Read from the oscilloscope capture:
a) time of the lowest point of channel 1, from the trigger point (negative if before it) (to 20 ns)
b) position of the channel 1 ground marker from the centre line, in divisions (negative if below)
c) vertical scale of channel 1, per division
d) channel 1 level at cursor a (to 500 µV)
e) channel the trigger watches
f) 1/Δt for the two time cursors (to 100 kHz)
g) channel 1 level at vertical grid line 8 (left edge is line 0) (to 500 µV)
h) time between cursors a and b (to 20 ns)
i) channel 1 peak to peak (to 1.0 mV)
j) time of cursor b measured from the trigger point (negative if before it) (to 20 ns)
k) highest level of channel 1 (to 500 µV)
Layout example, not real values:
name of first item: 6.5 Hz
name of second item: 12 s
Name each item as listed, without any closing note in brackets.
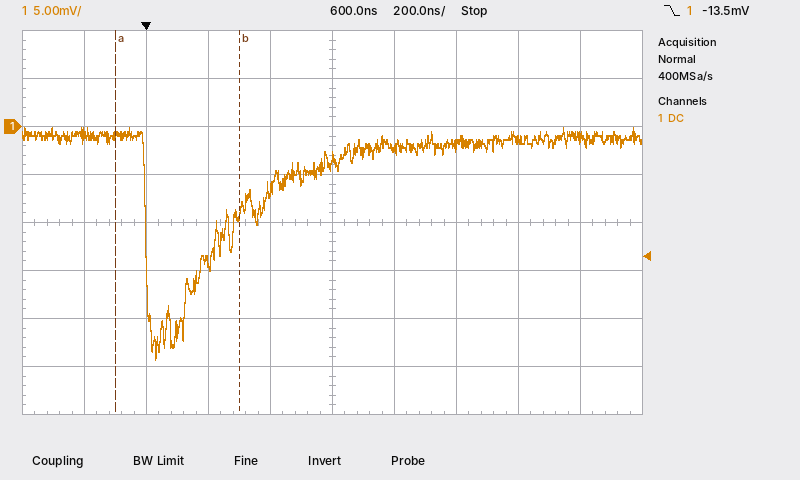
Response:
time of the lowest point of channel 1, from the trigger point (negative if before it): +40 ns
position of the channel 1 ground marker from the centre line, in divisions: +2.0 div
vertical scale of channel 1, per division: 5 mV
channel 1 level at cursor a: -1.0 mV
channel the trigger watches: channel 1
1/Δt for the two time cursors: 2.5 MHz
channel 1 level at vertical grid line 8 (left edge is line 0): -1.5 mV
time between cursors a and b: 400 ns
channel 1 peak to peak: 24.0 mV
time of cursor b measured from the trigger point (negative if before it): +300 ns
highest level of channel 1: 0.0 mV
